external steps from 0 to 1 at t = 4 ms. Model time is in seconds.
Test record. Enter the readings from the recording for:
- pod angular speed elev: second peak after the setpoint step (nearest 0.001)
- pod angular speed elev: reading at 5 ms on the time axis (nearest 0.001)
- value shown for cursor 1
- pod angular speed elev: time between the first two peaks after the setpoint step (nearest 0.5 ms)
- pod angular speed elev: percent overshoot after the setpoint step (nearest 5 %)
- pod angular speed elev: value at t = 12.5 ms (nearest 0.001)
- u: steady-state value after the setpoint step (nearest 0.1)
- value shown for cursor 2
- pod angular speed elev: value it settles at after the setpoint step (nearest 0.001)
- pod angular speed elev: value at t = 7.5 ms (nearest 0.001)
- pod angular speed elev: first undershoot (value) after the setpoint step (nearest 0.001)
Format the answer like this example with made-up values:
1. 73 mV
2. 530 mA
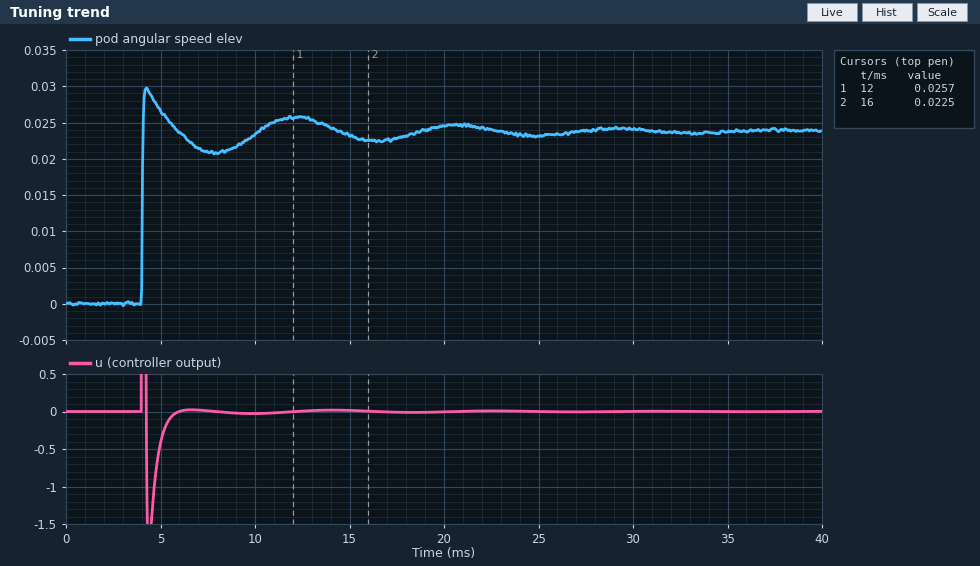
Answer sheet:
1. 0.026
2. 0.027
3. 0.0257
4. 8.0 ms
5. 25 %
6. 0.026
7. 0.0
8. 0.0225
9. 0.024
10. 0.021
11. 0.021
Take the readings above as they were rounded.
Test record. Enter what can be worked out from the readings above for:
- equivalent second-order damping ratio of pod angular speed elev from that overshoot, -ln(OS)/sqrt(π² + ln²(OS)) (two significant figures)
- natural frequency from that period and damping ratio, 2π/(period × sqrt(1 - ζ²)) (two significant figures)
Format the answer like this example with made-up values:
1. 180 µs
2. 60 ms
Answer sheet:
1. 0.40
2. 0.86 rad/ms
